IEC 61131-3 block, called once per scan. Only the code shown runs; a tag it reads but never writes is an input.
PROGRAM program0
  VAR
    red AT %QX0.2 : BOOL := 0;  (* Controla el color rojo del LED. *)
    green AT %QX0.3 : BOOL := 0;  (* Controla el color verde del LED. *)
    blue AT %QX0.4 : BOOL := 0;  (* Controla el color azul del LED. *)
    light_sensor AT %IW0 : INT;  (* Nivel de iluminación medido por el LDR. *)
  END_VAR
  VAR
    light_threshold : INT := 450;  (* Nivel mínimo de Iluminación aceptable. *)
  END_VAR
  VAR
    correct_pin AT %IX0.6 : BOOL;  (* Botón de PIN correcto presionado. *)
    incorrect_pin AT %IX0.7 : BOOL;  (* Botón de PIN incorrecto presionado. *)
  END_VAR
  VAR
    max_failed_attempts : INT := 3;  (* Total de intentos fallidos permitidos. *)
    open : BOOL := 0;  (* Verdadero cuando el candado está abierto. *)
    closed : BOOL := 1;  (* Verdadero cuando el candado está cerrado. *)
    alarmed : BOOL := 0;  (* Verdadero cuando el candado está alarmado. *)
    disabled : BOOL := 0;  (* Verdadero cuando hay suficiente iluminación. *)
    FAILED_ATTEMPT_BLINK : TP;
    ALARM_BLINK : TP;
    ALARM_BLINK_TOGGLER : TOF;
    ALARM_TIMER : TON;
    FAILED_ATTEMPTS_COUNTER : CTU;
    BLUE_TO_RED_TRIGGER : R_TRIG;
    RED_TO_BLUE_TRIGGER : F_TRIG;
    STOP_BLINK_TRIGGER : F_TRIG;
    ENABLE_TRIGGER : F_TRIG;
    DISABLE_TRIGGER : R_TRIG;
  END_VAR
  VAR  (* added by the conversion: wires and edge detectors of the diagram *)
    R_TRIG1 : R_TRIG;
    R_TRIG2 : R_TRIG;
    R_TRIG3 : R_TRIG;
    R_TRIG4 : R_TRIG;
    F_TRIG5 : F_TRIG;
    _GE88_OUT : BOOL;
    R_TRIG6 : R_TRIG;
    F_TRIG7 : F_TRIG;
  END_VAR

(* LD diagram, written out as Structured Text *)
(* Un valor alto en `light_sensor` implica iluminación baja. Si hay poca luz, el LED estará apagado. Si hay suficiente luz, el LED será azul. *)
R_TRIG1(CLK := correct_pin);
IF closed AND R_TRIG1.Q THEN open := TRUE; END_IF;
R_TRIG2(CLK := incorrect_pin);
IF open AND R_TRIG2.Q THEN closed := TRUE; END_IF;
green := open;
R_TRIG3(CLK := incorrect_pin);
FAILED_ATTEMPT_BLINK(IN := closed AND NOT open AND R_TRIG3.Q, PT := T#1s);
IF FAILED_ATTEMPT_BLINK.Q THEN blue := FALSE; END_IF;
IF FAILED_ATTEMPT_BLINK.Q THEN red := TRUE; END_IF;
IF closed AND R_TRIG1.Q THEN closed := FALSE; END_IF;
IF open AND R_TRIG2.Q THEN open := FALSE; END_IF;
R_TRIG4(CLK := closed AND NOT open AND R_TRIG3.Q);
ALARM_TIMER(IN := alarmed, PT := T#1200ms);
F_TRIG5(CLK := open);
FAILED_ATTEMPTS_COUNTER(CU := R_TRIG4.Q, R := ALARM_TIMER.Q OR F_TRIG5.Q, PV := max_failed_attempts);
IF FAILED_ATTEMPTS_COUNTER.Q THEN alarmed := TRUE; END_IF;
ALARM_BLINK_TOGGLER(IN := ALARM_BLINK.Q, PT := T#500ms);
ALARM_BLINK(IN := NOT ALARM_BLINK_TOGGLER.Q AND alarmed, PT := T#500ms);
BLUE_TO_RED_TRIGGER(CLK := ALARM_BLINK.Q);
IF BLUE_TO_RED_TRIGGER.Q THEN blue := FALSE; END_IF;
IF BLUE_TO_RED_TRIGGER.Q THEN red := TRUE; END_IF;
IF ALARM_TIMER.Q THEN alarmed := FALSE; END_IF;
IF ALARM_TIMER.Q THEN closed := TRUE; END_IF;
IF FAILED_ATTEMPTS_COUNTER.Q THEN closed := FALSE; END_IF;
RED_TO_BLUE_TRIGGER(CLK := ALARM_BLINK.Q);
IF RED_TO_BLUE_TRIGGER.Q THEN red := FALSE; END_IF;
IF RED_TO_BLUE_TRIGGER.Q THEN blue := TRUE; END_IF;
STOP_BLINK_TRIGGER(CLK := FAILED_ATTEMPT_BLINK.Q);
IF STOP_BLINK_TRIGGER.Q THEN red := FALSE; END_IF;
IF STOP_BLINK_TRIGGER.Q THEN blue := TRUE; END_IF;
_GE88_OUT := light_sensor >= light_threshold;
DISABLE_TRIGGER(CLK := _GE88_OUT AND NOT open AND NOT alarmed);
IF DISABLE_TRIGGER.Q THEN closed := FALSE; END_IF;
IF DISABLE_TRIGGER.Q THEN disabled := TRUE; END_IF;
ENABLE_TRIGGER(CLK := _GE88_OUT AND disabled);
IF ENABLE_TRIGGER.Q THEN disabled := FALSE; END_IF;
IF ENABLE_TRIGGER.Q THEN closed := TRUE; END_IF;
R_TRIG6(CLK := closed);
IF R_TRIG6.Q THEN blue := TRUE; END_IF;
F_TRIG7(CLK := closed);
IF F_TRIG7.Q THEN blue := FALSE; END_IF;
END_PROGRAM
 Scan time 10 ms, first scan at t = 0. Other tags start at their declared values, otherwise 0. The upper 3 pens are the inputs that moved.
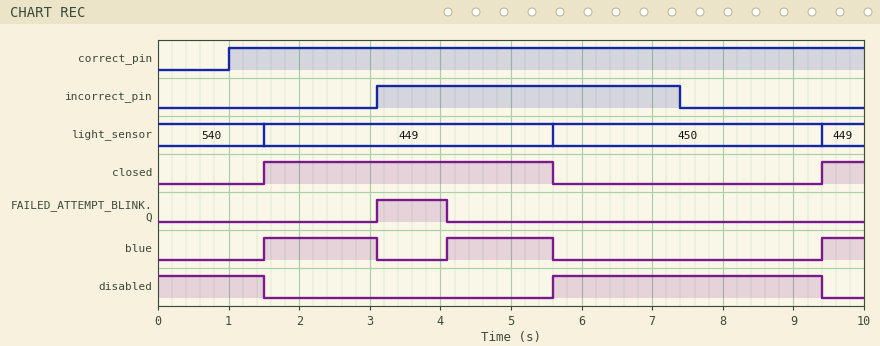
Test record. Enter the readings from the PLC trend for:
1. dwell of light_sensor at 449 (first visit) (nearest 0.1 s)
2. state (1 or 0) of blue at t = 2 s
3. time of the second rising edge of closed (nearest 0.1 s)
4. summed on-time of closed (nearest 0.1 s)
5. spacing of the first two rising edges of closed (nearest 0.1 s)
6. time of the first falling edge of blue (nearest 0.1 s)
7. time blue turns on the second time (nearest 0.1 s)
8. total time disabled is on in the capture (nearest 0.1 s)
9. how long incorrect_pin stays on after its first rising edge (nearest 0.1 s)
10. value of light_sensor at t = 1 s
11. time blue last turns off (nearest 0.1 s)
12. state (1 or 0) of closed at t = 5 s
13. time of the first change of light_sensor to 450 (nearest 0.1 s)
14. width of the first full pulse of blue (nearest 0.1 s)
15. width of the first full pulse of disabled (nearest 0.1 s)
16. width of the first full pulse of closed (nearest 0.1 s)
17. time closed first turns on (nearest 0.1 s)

4.1 s
1
9.4 s
4.7 s
7.9 s
3.1 s
4.1 s
5.3 s
4.3 s
540
5.6 s
1
5.6 s
1.6 s
3.8 s
4.1 s
1.5 s
